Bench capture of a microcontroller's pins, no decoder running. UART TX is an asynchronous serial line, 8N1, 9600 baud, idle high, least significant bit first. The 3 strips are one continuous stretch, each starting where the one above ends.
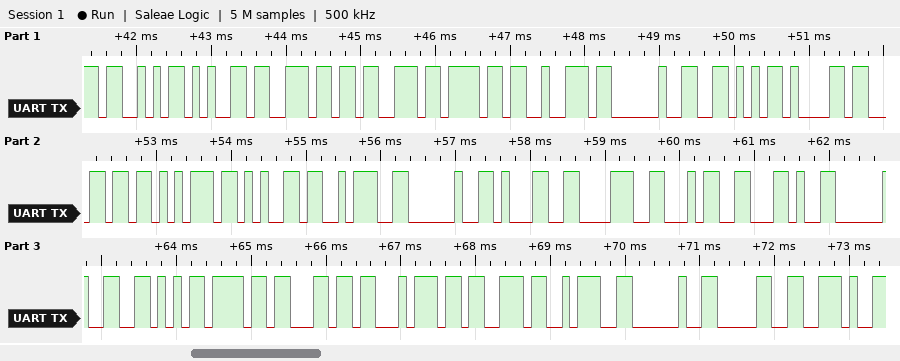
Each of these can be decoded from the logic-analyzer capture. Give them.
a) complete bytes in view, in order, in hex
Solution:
0x53 0x65 0x6E 0x73 0x6F 0x72 0x20 0x56 0x61 0x6C 0x75 0x65 0x3A 0x20 0x31 0x38 0x34 0x2C 0x20 0x56 0x6F 0x6C 0x74 0x73 0x3A 0x20 0x30 0x2E
